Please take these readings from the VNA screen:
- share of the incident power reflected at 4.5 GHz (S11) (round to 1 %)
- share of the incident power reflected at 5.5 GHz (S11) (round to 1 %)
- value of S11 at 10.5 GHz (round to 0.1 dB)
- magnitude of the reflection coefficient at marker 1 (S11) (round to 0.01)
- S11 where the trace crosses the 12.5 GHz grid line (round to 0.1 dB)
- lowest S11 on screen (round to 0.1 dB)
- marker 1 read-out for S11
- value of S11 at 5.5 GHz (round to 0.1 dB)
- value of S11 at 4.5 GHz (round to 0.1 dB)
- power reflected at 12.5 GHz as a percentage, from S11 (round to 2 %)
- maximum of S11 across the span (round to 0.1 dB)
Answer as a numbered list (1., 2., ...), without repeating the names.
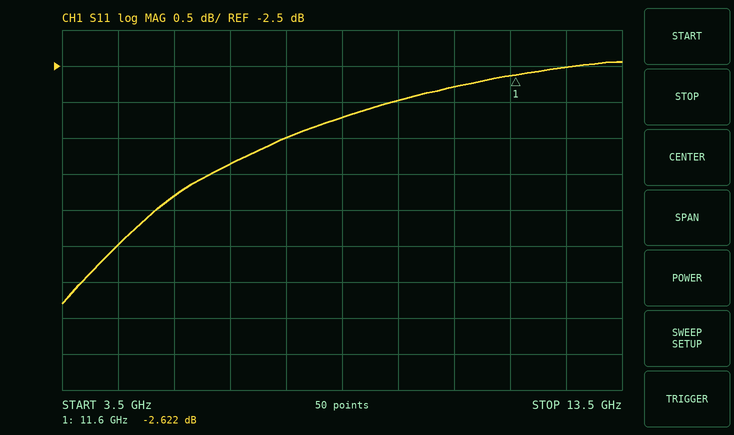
1. 32 %
2. 37 %
3. -2.8 dB
4. 0.74
5. -2.5 dB
6. -5.8 dB
7. -2.622 dB
8. -4.3 dB
9. -5.0 dB
10. 56 %
11. -2.4 dB
